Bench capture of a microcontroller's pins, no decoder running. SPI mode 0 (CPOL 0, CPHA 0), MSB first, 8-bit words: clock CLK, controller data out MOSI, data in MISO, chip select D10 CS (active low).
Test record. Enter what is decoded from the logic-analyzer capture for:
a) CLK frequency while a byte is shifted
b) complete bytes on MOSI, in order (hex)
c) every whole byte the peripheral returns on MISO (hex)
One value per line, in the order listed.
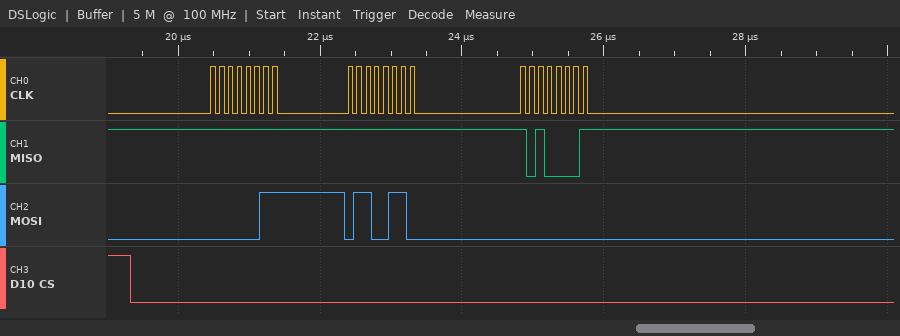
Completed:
8 MHz
03 66 00
FF FF A1
